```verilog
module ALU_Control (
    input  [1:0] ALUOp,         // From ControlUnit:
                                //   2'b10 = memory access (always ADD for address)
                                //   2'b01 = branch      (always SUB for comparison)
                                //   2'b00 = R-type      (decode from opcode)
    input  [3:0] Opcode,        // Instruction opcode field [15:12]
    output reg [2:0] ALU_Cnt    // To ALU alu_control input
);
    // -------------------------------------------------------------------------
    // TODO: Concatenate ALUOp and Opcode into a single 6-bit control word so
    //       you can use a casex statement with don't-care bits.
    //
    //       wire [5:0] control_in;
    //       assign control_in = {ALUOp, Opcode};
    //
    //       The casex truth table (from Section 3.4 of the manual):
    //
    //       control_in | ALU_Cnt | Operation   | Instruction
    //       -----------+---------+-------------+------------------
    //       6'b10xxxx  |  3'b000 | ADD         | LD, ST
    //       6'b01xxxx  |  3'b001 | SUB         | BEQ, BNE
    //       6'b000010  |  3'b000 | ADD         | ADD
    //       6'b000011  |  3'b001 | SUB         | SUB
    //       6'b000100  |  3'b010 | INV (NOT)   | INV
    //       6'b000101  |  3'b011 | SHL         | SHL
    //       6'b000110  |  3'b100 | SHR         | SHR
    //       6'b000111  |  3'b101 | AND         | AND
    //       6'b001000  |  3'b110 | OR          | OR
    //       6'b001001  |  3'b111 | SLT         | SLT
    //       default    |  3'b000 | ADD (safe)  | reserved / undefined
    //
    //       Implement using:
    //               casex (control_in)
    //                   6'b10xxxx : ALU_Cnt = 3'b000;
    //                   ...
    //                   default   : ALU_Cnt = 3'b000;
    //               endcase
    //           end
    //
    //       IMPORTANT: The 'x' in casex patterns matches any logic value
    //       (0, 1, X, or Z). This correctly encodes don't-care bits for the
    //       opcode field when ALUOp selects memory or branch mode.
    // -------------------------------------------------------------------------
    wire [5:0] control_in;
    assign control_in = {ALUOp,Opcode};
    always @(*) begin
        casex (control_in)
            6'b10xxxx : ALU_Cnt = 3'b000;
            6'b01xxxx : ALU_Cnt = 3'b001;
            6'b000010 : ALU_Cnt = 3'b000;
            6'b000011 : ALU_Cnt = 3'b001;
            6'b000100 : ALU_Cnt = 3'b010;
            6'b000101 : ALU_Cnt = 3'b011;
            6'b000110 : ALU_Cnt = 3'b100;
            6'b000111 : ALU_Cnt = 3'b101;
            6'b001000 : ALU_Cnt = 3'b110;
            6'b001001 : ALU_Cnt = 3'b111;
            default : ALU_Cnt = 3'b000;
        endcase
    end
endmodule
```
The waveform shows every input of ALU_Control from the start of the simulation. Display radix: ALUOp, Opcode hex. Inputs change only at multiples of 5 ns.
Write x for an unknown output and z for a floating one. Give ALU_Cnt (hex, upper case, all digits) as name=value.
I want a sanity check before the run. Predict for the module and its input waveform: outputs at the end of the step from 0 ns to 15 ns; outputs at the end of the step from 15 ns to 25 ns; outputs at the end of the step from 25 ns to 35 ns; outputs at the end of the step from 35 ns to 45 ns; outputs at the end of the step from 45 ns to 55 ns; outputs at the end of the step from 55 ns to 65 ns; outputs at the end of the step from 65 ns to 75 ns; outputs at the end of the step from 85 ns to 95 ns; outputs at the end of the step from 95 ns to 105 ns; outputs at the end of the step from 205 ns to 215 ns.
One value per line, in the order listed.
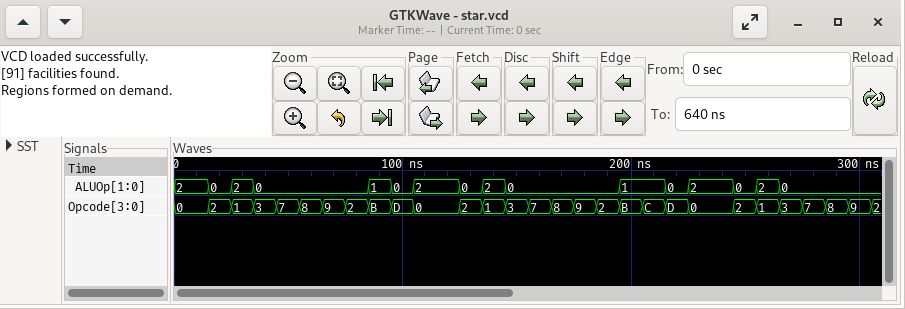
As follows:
ALU_Cnt=0
ALU_Cnt=0
ALU_Cnt=0
ALU_Cnt=1
ALU_Cnt=5
ALU_Cnt=6
ALU_Cnt=7
ALU_Cnt=1
ALU_Cnt=0
ALU_Cnt=1
